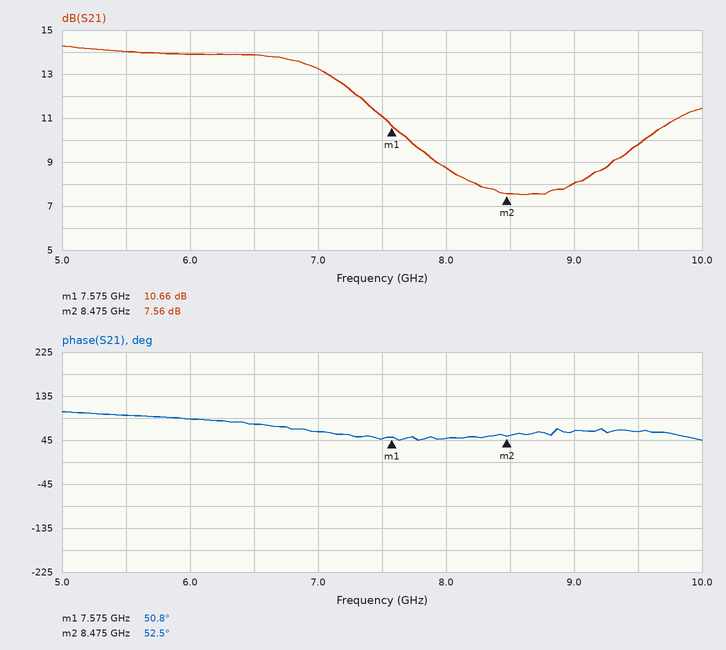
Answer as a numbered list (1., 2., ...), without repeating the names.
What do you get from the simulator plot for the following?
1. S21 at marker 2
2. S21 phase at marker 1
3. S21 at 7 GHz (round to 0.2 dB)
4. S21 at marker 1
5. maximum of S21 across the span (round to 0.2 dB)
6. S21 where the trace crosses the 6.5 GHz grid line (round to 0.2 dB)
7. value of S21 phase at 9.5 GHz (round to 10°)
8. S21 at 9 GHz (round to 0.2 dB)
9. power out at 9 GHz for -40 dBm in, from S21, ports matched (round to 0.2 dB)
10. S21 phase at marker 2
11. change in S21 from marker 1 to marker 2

1. 7.56 dB
2. 50.8°
3. 13.2 dB
4. 10.66 dB
5. 14.2 dB
6. 13.8 dB
7. 60°
8. 8.0 dB
9. -32.0 dBm
10. 52.5°
11. -3.10 dB
